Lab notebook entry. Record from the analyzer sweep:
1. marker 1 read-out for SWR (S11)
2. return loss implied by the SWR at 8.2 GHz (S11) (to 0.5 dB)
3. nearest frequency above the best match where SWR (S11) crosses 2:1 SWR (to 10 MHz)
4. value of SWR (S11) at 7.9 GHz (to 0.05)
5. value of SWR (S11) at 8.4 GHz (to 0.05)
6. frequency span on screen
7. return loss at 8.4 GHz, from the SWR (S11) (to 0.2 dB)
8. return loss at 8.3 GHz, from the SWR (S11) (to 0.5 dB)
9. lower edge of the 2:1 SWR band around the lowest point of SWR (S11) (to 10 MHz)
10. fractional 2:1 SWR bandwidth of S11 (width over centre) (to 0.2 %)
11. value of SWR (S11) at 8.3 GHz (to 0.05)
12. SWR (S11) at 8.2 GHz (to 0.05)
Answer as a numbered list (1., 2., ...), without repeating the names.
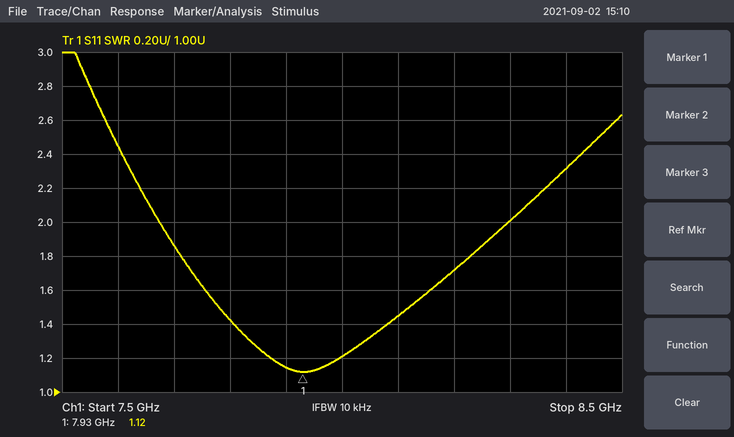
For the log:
1. 1.12
2. 11.5 dB
3. 8.30 GHz
4. 1.15
5. 2.30
6. 1 GHz
7. 8.0 dB
8. 9.5 dB
9. 7.67 GHz
10. 7.8 %
11. 2.00
12. 1.70
